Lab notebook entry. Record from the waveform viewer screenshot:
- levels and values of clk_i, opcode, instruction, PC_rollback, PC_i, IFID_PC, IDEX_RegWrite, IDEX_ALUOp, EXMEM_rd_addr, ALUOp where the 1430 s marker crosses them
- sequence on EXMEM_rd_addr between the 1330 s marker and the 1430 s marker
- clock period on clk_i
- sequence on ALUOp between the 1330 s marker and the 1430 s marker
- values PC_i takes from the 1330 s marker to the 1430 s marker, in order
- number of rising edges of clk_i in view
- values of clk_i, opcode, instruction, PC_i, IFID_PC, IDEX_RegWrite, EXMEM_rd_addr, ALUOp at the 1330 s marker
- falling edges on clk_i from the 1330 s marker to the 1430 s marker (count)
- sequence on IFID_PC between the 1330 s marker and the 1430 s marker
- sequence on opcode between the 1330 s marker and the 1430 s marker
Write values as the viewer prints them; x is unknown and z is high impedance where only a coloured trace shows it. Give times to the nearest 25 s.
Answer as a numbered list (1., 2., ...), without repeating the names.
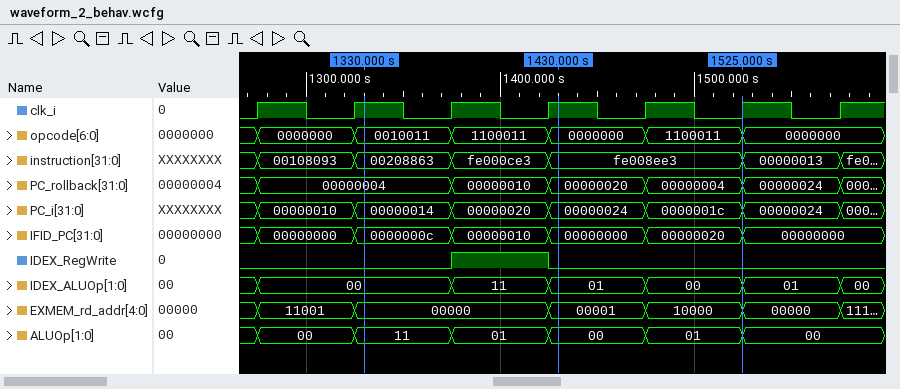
1. clk_i=1, opcode=0000000, instruction=fe008ee3, PC_rollback=00000020, PC_i=00000024, IFID_PC=00000000, IDEX_RegWrite=0, IDEX_ALUOp=01, EXMEM_rd_addr=00001, ALUOp=00
2. 00000, 00001
3. 50 s
4. 11, 01, 00
5. 00000014, 00000020, 00000024
6. 7
7. clk_i=1, opcode=0010011, instruction=00208863, PC_i=00000014, IFID_PC=0000000c, IDEX_RegWrite=0, EXMEM_rd_addr=00000, ALUOp=11
8. 2
9. 0000000c, 00000010, 00000000
10. 0010011, 1100011, 0000000
